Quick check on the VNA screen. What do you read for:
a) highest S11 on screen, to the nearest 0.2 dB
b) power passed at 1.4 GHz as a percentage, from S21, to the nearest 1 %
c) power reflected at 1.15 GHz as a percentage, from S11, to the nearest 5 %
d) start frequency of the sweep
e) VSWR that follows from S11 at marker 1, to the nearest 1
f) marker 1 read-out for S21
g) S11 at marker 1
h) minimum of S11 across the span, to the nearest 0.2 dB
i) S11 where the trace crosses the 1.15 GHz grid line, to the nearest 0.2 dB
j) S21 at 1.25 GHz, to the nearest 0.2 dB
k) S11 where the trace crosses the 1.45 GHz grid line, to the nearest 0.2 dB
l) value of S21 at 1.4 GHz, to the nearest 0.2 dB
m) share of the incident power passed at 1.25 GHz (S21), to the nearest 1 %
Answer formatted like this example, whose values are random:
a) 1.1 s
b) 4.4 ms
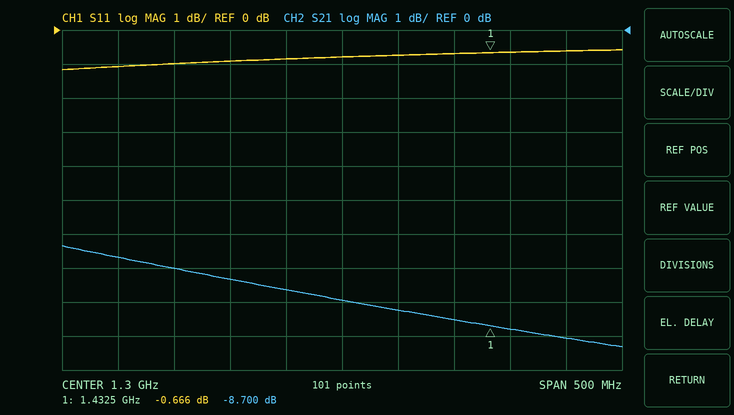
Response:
a) -0.6 dB
b) 14 %
c) 80 %
d) 1.05 GHz
e) 26
f) -8.700 dB
g) -0.666 dB
h) -1.2 dB
i) -1.0 dB
j) -7.6 dB
k) -0.6 dB
l) -8.6 dB
m) 17 %
